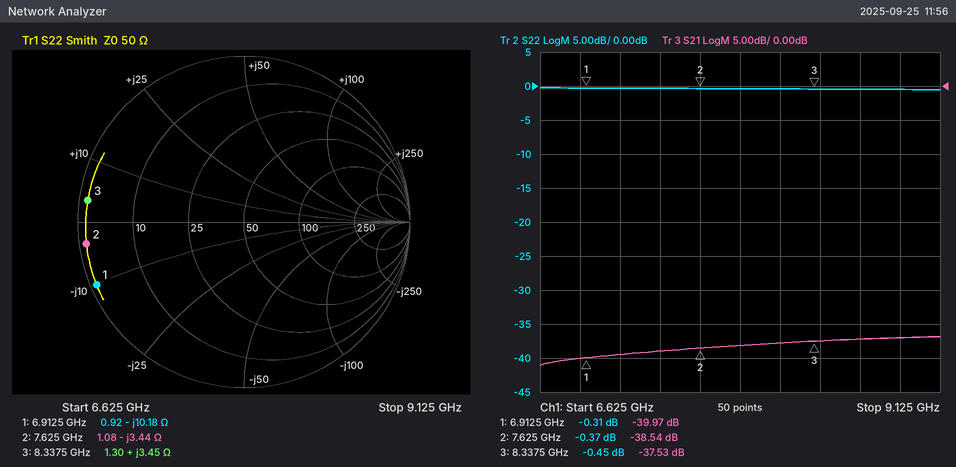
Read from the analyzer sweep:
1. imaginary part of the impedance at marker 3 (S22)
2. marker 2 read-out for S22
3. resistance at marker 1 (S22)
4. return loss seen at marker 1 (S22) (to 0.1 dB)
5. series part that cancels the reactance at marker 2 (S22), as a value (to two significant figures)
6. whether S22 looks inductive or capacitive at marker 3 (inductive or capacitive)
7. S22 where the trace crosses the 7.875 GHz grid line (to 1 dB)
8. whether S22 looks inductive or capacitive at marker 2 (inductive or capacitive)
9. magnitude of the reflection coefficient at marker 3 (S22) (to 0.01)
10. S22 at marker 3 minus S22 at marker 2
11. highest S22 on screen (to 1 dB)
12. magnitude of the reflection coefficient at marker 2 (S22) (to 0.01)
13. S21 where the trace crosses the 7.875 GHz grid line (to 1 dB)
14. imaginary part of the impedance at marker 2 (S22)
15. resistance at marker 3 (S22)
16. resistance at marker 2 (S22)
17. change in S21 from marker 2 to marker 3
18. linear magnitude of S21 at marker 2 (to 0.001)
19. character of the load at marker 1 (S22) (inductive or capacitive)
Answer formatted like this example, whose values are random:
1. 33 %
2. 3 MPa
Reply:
1. +3.45 Ω
2. -0.37 dB
3. 0.92 Ω
4. 0.3 dB
5. 72 pH
6. inductive
7. 0 dB
8. capacitive
9. 0.95
10. -0.08 dB
11. 0 dB
12. 0.96
13. -38 dB
14. -3.44 Ω
15. 1.30 Ω
16. 1.08 Ω
17. 1.01 dB
18. 0.012
19. capacitive
